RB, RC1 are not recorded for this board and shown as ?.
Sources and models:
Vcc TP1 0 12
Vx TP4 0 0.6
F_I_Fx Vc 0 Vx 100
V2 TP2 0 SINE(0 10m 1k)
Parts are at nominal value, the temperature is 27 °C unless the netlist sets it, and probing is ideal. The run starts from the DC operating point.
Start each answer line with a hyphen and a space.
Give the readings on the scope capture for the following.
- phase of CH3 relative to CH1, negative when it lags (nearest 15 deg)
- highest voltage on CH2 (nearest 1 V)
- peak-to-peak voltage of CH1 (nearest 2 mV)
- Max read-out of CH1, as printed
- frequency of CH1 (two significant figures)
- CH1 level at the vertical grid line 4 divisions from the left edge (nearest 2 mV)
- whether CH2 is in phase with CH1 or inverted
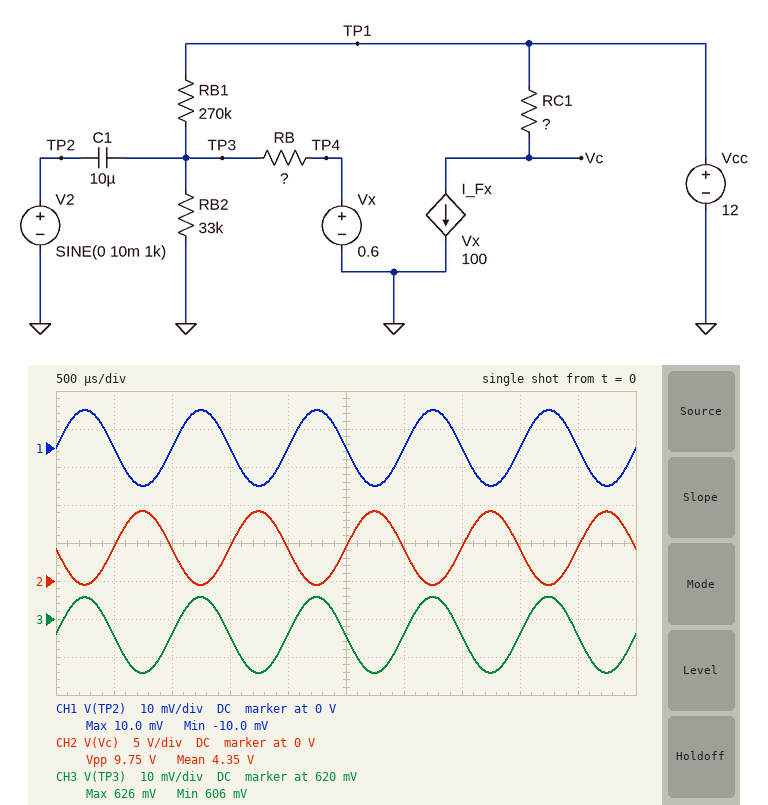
- 0 deg
- 9 V
- 20 mV
- 10.0 mV
- 1.0 kHz
- 0 V
- inverted
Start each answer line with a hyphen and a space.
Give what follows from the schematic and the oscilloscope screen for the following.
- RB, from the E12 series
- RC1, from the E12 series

- 680 Ω
- 3.3 kΩ
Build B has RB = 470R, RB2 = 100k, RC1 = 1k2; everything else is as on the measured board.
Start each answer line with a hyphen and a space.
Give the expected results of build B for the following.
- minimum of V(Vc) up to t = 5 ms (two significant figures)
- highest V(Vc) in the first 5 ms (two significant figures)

- 5.2 V
- 10 V
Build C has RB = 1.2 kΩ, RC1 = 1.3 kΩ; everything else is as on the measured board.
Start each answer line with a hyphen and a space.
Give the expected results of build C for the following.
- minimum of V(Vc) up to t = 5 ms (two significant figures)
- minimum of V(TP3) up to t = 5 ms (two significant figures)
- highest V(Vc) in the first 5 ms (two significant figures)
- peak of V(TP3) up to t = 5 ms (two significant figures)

- 7.9 V
- 620 mV
- 10 V
- 640 mV
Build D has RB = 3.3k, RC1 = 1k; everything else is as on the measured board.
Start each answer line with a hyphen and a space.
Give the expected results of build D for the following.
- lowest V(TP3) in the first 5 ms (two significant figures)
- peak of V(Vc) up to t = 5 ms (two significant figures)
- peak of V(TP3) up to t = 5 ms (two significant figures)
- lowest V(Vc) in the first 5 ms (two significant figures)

- 660 mV
- 10 V
- 680 mV
- 9.5 V
